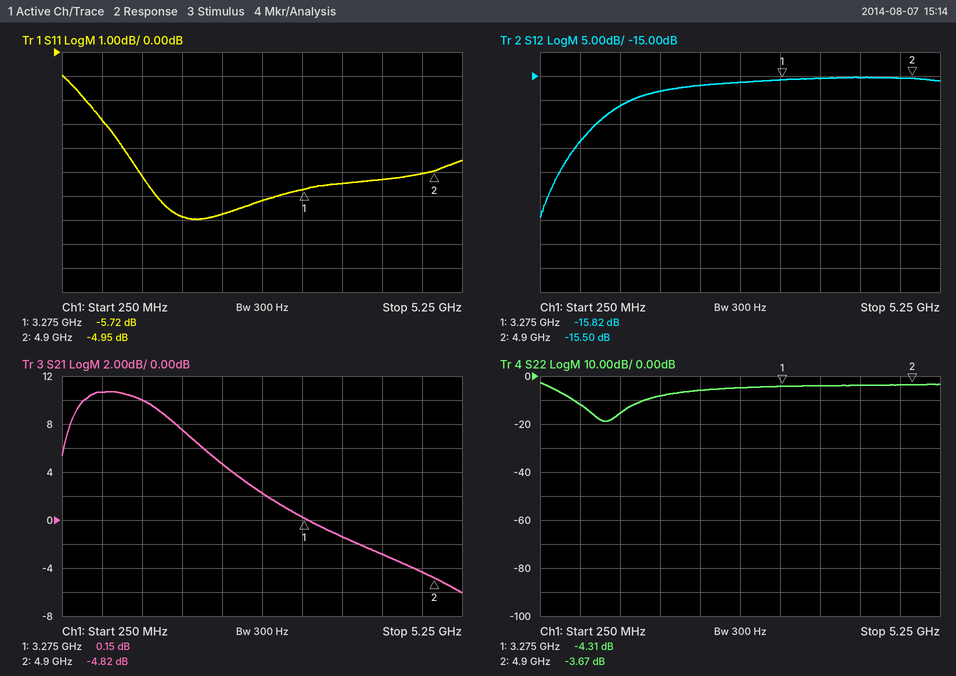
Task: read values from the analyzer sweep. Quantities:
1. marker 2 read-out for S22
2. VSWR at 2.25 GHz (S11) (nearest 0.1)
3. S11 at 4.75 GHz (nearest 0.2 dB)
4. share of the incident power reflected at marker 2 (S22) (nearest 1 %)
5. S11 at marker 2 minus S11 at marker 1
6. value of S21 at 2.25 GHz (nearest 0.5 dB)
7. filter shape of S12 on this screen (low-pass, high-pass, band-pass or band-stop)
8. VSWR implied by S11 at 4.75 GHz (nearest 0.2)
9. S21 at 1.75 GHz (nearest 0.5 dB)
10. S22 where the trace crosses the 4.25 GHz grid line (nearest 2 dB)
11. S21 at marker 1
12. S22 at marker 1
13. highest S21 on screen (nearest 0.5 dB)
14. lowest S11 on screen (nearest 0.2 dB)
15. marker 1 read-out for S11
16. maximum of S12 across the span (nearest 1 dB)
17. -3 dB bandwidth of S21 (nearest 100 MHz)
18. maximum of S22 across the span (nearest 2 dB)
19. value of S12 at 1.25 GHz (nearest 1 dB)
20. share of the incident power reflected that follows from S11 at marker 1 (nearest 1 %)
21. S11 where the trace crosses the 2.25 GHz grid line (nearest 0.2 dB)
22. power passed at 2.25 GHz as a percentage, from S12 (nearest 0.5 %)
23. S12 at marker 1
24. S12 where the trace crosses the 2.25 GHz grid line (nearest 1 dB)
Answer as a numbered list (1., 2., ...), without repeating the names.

1. -3.67 dB
2. 2.7
3. -5.0 dB
4. 43 %
5. 0.77 dB
6. 4.5 dB
7. high-pass
8. 3.6
9. 7.5 dB
10. -4 dB
11. 0.15 dB
12. -4.31 dB
13. 10.5 dB
14. -7.0 dB
15. -5.72 dB
16. -15 dB
17. 1.4 GHz
18. -2 dB
19. -21 dB
20. 27 %
21. -6.8 dB
22. 2.0 %
23. -15.82 dB
24. -17 dB
